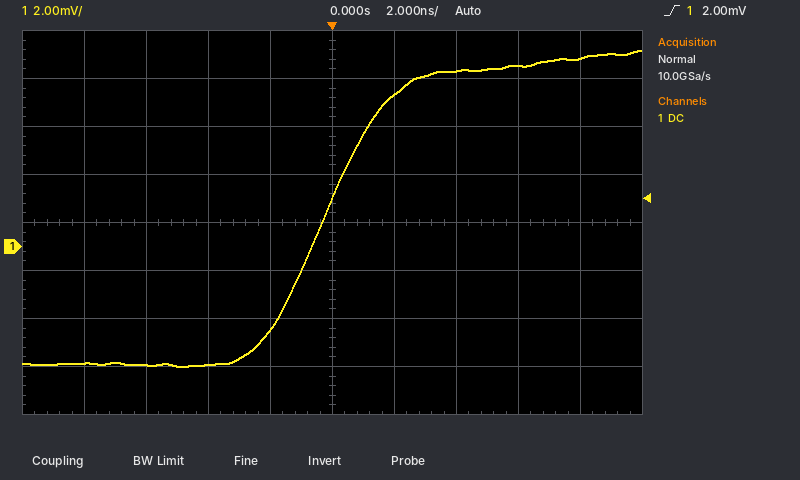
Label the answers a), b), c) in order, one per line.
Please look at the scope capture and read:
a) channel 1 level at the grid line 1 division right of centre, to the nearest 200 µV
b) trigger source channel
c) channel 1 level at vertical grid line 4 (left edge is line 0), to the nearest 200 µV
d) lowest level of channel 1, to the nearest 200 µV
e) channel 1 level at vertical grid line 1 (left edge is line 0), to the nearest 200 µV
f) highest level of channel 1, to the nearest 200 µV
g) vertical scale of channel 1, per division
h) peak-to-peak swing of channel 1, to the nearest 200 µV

a) 6.4 mV
b) channel 1
c) -3.4 mV
d) -5.0 mV
e) -4.8 mV
f) 8.2 mV
g) 2 mV
h) 13.2 mV
